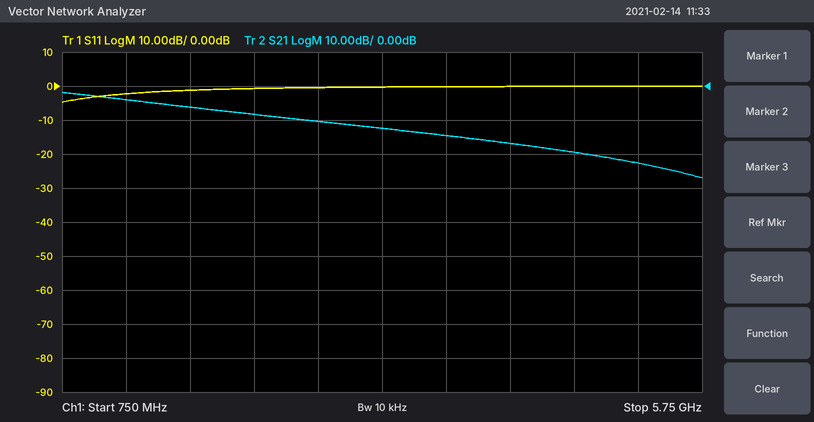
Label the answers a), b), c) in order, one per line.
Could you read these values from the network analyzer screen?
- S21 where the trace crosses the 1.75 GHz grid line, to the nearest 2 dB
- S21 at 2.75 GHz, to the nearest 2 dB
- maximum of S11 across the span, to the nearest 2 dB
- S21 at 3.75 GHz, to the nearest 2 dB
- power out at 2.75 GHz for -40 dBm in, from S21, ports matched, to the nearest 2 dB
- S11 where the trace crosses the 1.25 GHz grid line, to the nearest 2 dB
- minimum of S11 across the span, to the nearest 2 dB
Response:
a) -6 dB
b) -10 dB
c) 0 dB
d) -14 dB
e) -50 dBm
f) -2 dB
g) -4 dB
